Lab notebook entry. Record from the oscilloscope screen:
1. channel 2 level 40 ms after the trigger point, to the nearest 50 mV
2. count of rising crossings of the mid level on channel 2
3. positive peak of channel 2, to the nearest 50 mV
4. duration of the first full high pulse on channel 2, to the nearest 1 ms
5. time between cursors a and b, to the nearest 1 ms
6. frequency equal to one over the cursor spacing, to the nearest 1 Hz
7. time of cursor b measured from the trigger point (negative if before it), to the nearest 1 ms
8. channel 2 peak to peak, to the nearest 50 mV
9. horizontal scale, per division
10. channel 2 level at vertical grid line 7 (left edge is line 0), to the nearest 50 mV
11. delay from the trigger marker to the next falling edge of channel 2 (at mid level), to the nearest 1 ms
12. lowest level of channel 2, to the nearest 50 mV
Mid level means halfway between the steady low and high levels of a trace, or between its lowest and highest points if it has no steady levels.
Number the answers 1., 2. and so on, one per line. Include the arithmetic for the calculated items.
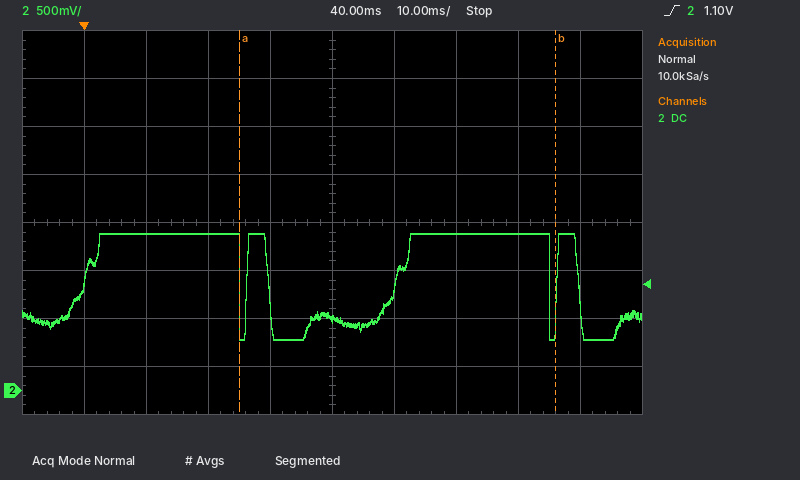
1. 750 mV
2. 4
3. 1.65 V
4. 25 ms
5. 51 ms
6. 1 / 51 ms ≈ 20 Hz
7. +76 ms
8. 1.65 V − (550 mV) = 1.10 V
9. 10 ms
10. 1.65 V
11. 25 ms
12. 550 mV
